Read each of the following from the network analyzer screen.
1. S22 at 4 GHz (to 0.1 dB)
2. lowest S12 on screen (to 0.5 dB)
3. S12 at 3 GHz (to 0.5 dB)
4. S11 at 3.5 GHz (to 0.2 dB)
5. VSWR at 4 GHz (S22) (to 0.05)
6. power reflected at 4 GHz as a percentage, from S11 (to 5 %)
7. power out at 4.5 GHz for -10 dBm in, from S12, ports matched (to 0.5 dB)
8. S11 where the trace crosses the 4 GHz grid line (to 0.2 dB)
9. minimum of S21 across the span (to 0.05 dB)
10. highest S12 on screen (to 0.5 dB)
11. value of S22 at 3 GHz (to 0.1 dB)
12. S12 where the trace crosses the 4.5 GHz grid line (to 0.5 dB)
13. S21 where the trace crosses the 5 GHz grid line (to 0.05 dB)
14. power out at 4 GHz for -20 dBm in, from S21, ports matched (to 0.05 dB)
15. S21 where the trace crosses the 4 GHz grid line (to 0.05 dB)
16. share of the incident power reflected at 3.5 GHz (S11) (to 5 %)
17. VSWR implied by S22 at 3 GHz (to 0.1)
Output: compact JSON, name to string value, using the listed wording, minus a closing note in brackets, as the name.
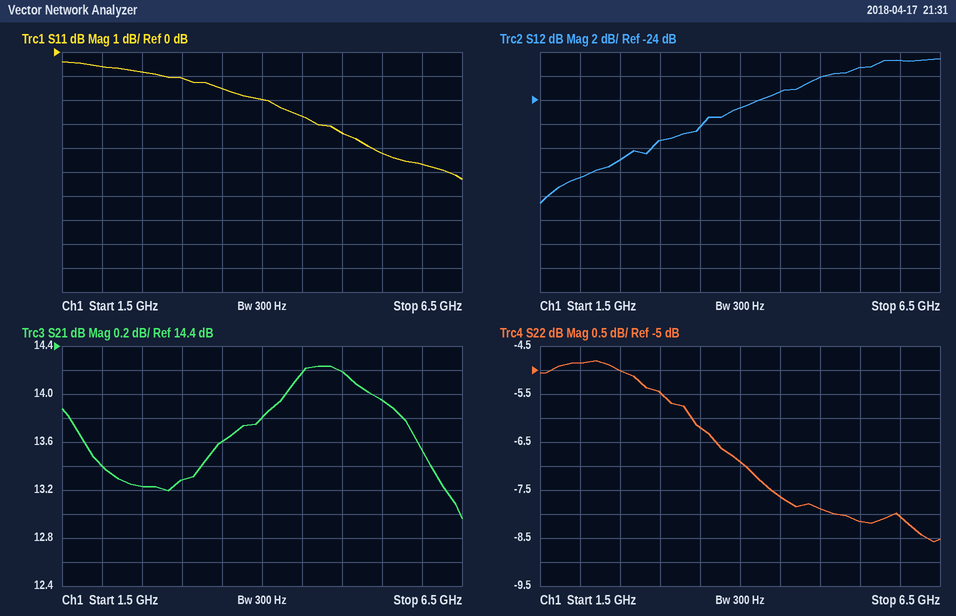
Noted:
{"S22 at 4 GHz": "-6.9 dB", "lowest S12 on screen": "-32.5 dB", "S12 at 3 GHz": "-27.5 dB", "S11 at 3.5 GHz": "-1.6 dB", "VSWR at 4 GHz (S22)": "2.65", "power reflected at 4 GHz as a percentage, from S11": "65 %", "power out at 4.5 GHz for -10 dBm in, from S12, ports matched": "-33.5 dBm", "S11 where the trace crosses the 4 GHz grid line": "-2.0 dB", "minimum of S21 across the span": "12.95 dB", "highest S12 on screen": "-20.5 dB", "value of S22 at 3 GHz": "-5.5 dB", "S12 where the trace crosses the 4.5 GHz grid line": "-23.5 dB", "S21 where the trace crosses the 5 GHz grid line": "14.20 dB", "power out at 4 GHz for -20 dBm in, from S21, ports matched": "-6.20 dBm", "S21 where the trace crosses the 4 GHz grid line": "13.80 dB", "share of the incident power reflected at 3.5 GHz (S11)": "70 %", "VSWR implied by S22 at 3 GHz": "3.3"}
